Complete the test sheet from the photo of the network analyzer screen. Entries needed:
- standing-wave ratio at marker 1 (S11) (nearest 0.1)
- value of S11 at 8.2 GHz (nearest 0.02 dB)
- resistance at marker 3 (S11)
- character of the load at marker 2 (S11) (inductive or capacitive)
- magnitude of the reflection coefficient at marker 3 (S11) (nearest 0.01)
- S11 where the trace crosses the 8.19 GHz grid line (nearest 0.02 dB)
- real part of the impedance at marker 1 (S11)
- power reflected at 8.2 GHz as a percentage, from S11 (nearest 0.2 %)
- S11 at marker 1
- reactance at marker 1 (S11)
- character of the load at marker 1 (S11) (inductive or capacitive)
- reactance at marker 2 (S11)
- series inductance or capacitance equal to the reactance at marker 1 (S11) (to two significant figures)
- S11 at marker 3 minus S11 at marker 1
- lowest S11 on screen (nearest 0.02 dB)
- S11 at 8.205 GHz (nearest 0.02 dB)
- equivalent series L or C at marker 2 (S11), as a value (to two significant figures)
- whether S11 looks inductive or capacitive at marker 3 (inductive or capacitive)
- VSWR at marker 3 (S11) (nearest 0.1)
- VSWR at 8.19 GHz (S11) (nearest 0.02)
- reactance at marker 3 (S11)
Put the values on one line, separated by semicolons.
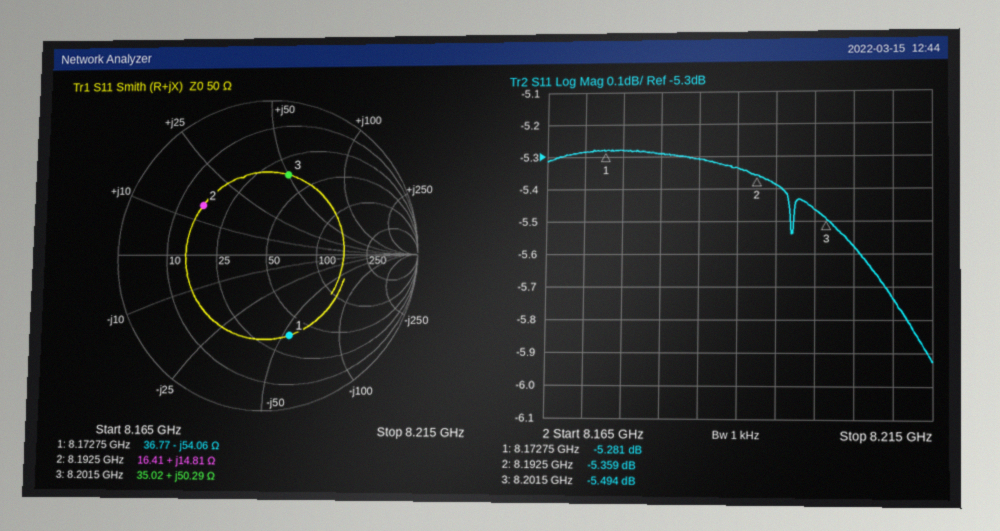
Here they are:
3.4; -5.46 dB; 35.02 Ω; inductive; 0.53; -5.34 dB; 36.77 Ω; 28.4 %; -5.281 dB; -54.06 Ω; capacitive; +14.81 Ω; 360 fF; -0.213 dB; -5.92 dB; -5.58 dB; 290 pH; inductive; 3.3; 3.36; +50.29 Ω
